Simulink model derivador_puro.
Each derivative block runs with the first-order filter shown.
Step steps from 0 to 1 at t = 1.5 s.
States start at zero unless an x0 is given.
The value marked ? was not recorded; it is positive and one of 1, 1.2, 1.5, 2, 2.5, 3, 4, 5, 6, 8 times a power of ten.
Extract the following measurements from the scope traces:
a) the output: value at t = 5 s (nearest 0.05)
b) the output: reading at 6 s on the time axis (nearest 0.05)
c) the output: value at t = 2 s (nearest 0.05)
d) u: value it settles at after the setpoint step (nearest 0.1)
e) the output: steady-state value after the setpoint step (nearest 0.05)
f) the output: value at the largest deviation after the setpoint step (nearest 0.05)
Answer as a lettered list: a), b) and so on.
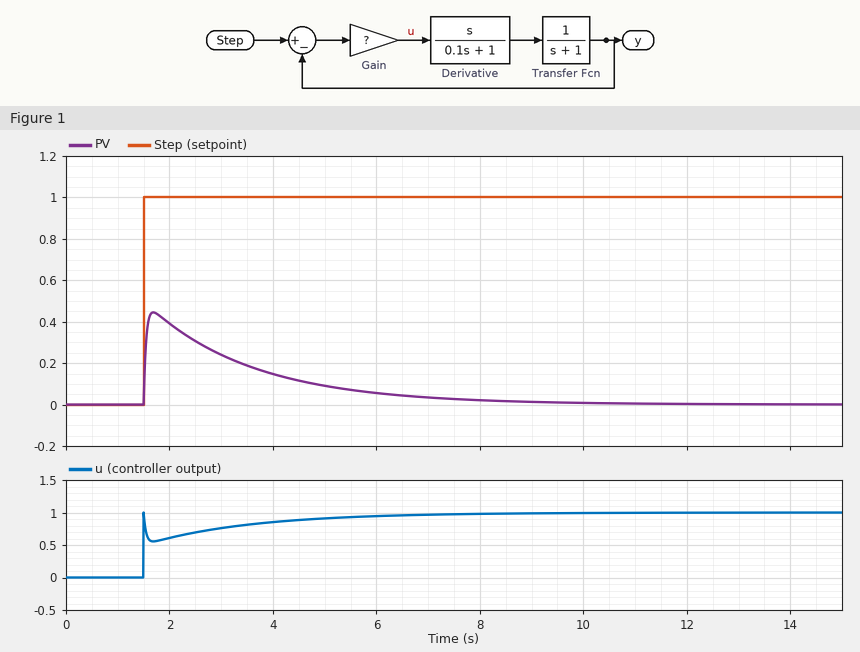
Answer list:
a) 0.10
b) 0.05
c) 0.40
d) 1.0
e) 0.00
f) 0.45
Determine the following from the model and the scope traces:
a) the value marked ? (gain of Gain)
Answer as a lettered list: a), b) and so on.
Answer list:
a) 1
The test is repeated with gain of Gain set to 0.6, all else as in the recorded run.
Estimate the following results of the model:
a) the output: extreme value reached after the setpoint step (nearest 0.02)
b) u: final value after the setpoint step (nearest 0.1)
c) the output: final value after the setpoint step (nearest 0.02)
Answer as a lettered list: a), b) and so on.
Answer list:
a) 0.32
b) 0.6
c) 0.00
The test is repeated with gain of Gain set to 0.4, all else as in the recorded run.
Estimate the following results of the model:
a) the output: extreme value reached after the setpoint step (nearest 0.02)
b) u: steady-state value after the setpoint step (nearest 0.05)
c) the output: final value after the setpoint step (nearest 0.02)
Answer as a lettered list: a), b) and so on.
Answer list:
a) 0.24
b) 0.40
c) 0.00
